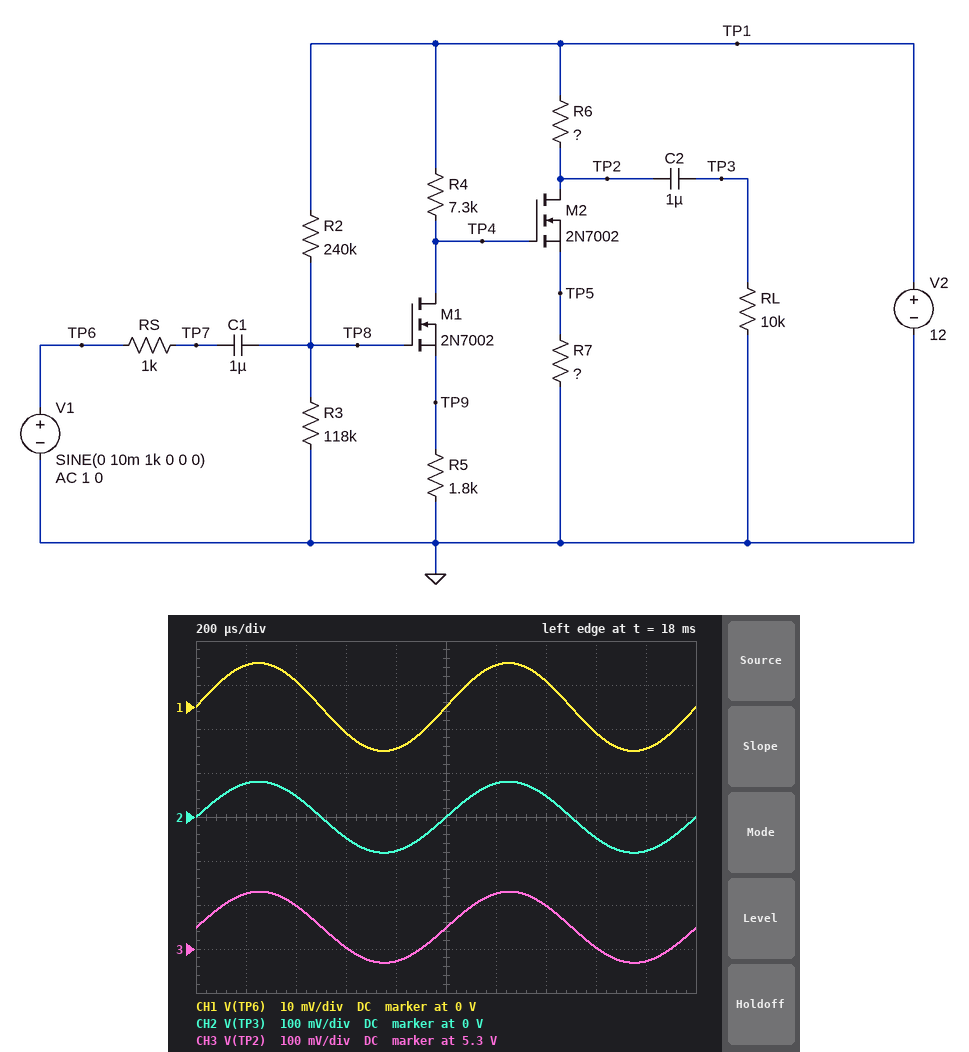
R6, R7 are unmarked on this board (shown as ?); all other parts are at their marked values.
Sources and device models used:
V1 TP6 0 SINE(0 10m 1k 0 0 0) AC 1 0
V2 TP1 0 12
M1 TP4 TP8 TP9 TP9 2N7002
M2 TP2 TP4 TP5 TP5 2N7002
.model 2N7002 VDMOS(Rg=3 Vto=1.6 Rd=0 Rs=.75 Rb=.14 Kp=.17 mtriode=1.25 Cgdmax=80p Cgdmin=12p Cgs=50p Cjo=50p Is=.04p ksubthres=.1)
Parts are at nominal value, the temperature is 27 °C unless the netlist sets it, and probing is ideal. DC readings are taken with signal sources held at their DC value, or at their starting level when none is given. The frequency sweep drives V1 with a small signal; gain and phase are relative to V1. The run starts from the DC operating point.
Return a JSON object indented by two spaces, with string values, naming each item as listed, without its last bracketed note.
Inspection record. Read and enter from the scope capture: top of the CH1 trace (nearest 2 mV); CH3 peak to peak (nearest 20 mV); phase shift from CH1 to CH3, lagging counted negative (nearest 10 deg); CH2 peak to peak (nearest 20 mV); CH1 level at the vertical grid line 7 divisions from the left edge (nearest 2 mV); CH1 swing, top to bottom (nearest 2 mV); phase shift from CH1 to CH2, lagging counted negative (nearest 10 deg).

{
  "top of the CH1 trace": "10 mV",
  "CH3 peak to peak": "160 mV",
  "phase shift from CH1 to CH3, lagging counted negative": "0 deg",
  "CH2 peak to peak": "160 mV",
  "CH1 level at the vertical grid line 7 divisions from the left edge": "6 mV",
  "CH1 swing, top to bottom": "20 mV",
  "phase shift from CH1 to CH2, lagging counted negative": "0 deg"
}
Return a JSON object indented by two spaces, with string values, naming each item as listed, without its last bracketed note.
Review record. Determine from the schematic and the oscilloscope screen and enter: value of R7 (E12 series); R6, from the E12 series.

{
  "value of R7": "2.7 kΩ",
  "R6, from the E12 series": "15 kΩ"
}
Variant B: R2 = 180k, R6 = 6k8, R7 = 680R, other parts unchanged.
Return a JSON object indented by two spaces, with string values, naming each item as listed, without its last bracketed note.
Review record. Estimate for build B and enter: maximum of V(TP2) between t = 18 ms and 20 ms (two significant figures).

{
  "maximum of V(TP2) between t = 18 ms and 20 ms": "4.9 V"
}
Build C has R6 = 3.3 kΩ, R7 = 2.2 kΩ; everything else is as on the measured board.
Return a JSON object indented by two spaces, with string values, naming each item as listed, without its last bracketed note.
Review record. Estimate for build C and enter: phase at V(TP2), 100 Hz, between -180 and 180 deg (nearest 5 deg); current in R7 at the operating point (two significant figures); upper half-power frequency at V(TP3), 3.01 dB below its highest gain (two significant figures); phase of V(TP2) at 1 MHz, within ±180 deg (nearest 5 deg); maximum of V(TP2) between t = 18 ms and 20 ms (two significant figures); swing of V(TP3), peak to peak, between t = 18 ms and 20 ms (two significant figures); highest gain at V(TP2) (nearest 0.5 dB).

{
  "phase at V(TP2), 100 Hz, between -180 and 180 deg": "0 deg",
  "current in R7 at the operating point": "540 µA",
  "upper half-power frequency at V(TP3), 3.01 dB below its highest gain": "140 kHz",
  "phase of V(TP2) at 1 MHz, within ±180 deg": "-160 deg",
  "maximum of V(TP2) between t = 18 ms and 20 ms": "10 V",
  "swing of V(TP3), peak to peak, between t = 18 ms and 20 ms": "82 mV",
  "highest gain at V(TP2)": "14.0 dB"
}
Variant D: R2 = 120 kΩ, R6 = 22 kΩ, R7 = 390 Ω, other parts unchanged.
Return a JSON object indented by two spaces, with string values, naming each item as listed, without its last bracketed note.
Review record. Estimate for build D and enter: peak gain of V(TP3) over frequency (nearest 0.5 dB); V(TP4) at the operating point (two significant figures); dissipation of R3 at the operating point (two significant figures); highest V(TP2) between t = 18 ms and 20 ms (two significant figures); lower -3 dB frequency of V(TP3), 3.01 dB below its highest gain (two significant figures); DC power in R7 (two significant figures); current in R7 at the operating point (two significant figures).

{
  "peak gain of V(TP3) over frequency": "-13.0 dB",
  "V(TP4) at the operating point": "2.4 V",
  "dissipation of R3 at the operating point": "300 µW",
  "highest V(TP2) between t = 18 ms and 20 ms": "210 mV",
  "lower -3 dB frequency of V(TP3), 3.01 dB below its highest gain": "1.9 MHz",
  "DC power in R7": "110 µW",
  "current in R7 at the operating point": "540 µA"
}
